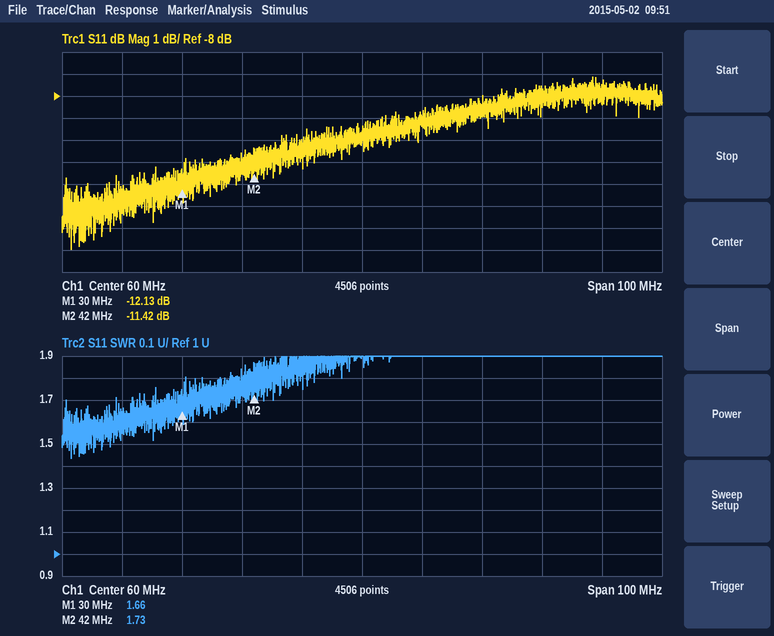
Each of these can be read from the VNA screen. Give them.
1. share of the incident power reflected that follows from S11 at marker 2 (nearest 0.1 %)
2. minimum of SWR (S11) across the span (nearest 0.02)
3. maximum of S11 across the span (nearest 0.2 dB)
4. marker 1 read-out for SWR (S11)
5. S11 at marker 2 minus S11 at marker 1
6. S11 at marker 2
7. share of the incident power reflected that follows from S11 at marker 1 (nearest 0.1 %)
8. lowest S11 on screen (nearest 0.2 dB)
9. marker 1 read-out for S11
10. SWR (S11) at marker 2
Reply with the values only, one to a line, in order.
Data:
7.2 %
1.44
-7.2 dB
1.66
0.71 dB
-11.42 dB
6.1 %
-15.0 dB
-12.13 dB
1.73
